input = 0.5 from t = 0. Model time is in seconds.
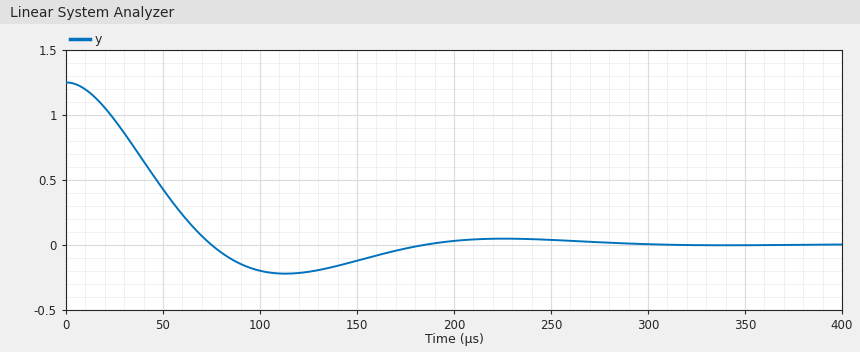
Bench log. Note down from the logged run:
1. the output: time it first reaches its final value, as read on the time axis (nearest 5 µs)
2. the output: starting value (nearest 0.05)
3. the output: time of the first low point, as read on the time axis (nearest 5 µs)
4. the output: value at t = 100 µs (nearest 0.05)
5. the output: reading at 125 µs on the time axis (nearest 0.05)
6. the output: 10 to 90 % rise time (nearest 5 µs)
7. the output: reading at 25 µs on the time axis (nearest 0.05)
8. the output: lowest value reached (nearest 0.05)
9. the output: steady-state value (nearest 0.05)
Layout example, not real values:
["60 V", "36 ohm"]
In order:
["75 µs", "1.25", "115 µs", "-0.20", "-0.20", "50 µs", "0.95", "-0.20", "0.00"]
